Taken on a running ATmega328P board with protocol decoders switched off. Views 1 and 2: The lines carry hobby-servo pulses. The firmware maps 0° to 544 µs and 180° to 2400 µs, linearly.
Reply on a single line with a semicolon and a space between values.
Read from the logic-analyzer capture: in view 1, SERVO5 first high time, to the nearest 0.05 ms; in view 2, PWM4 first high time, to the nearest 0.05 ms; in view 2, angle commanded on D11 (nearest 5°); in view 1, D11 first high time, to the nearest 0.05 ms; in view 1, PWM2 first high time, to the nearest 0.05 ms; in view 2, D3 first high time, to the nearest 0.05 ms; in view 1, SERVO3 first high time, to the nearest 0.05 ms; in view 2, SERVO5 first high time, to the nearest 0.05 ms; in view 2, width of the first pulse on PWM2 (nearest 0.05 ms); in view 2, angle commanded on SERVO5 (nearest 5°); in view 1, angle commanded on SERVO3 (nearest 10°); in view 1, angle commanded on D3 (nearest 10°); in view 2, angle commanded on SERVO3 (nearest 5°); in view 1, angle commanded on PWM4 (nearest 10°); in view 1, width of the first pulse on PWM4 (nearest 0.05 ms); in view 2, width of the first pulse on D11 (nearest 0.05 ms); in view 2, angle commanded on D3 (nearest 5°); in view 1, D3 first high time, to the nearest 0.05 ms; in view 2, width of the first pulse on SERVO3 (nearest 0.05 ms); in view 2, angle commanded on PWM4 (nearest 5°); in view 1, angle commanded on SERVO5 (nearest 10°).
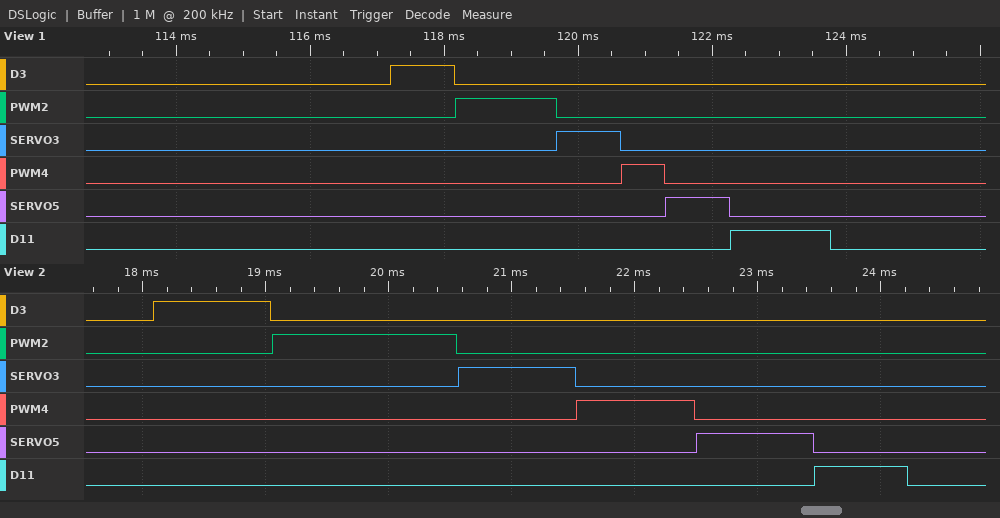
0.95 ms; 0.95 ms; 20°; 1.50 ms; 1.50 ms; 0.95 ms; 0.95 ms; 0.95 ms; 1.50 ms; 40°; 40°; 40°; 40°; 10°; 0.65 ms; 0.75 ms; 40°; 0.95 ms; 0.95 ms; 40°; 40°
